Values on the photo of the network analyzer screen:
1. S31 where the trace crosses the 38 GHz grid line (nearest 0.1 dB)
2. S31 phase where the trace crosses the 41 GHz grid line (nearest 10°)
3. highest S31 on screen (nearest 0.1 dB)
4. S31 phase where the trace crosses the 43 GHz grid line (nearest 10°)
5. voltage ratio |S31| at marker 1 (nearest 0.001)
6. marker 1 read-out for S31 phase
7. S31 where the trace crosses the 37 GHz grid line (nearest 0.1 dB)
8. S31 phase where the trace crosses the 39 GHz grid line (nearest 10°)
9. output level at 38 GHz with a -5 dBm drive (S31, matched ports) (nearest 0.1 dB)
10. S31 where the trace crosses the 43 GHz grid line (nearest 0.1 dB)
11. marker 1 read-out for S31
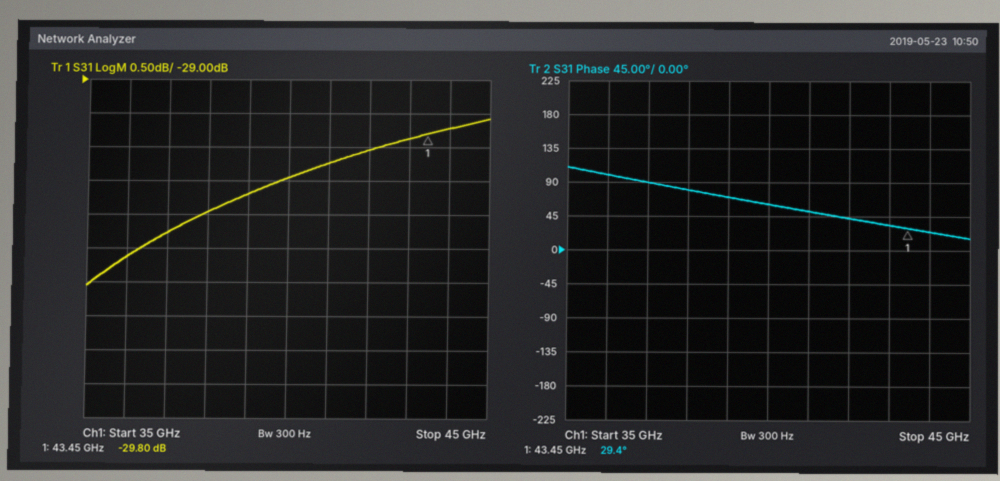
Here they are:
-31.0 dB
50°
-29.6 dB
30°
0.032
29.4°
-31.3 dB
70°
-36.0 dBm
-29.9 dB
-29.80 dB
